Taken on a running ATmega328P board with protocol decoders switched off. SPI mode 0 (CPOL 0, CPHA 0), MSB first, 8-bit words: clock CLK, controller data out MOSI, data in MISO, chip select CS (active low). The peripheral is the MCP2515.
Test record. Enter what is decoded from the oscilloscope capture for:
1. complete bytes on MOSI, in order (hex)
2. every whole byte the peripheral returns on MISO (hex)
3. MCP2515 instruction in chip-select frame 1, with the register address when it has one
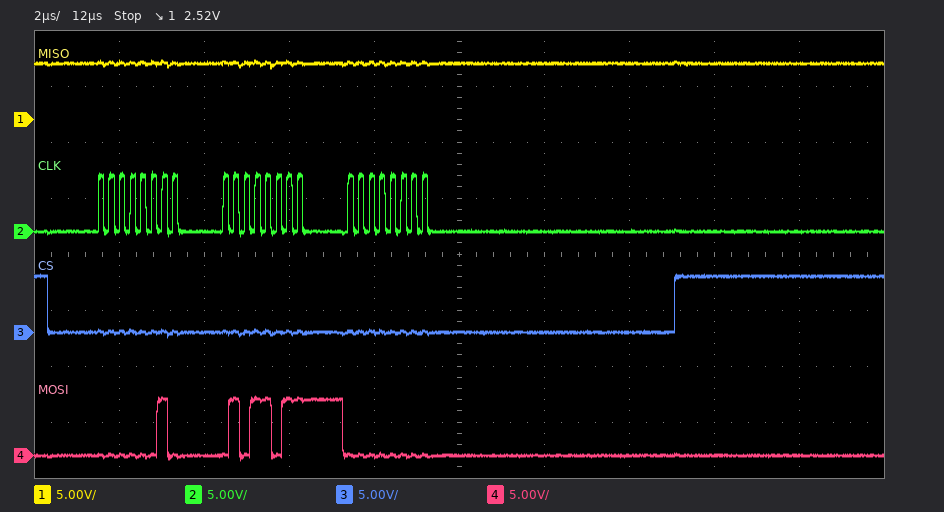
0x02 0x5B 0x00
0xFF 0xFF 0xFF
WRITE 0x5B
